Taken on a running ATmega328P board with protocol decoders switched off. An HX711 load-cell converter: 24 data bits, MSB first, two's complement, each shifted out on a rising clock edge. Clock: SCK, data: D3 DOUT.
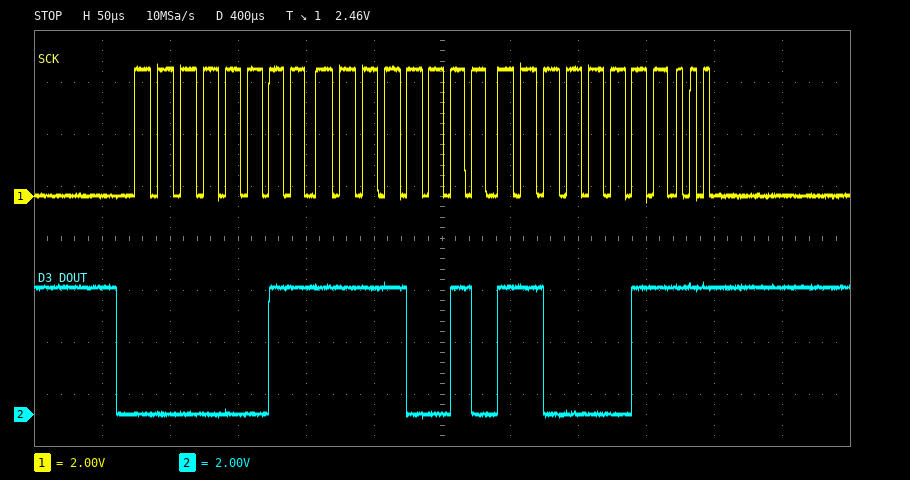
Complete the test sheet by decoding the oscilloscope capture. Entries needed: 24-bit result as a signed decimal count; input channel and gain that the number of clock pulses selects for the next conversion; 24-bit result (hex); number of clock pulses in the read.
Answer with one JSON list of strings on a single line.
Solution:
["258755", "channel A, gain 64", "0x03F2C3", "27"]
